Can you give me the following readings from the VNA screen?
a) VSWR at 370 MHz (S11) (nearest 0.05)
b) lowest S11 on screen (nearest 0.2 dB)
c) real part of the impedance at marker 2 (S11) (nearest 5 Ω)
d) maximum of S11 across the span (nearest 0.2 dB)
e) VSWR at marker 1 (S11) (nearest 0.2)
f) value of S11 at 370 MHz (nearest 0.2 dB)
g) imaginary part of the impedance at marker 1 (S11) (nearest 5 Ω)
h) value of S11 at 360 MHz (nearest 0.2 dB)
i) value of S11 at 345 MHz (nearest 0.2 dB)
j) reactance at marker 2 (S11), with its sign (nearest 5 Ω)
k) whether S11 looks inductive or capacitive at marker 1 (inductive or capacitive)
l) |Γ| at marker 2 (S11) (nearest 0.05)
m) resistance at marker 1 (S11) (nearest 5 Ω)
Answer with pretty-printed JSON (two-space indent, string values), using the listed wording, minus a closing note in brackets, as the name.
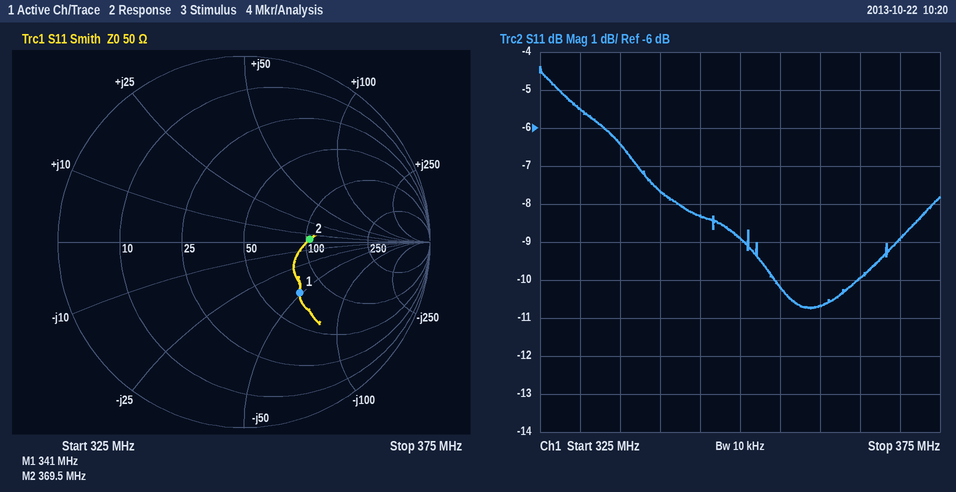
{
  "VSWR at 370 MHz (S11)": "2.10",
  "lowest S11 on screen": "-10.8 dB",
  "real part of the impedance at marker 2 (S11)": "105 Ω",
  "maximum of S11 across the span": "-4.4 dB",
  "VSWR at marker 1 (S11)": "2.4",
  "value of S11 at 370 MHz": "-9.0 dB",
  "imaginary part of the impedance at marker 1 (S11)": "-50 Ω",
  "value of S11 at 360 MHz": "-10.6 dB",
  "value of S11 at 345 MHz": "-8.4 dB",
  "reactance at marker 2 (S11), with its sign": "+5 Ω",
  "whether S11 looks inductive or capacitive at marker 1": "capacitive",
  "|Γ| at marker 2 (S11)": "0.35",
  "resistance at marker 1 (S11)": "75 Ω"
}
